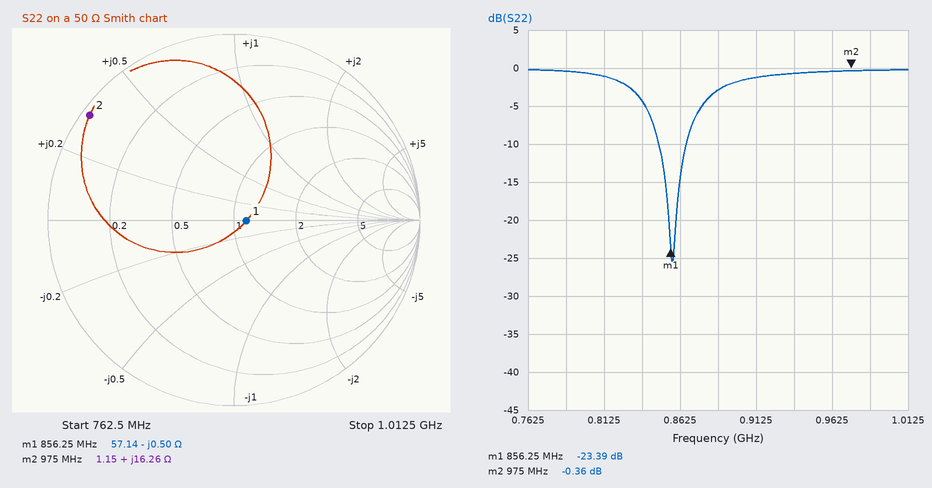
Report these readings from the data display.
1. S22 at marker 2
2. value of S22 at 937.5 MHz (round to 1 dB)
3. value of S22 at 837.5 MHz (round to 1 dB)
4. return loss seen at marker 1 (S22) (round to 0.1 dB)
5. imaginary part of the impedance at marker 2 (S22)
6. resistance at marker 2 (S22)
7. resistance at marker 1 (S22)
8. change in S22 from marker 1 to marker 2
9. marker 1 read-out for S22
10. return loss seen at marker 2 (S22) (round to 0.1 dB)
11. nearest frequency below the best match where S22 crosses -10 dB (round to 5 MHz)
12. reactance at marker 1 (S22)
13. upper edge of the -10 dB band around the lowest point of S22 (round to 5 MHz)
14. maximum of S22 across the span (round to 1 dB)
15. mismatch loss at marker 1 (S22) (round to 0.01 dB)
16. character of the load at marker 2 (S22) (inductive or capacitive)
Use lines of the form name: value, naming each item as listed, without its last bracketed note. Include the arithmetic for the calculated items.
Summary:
S22 at marker 2: -0.36 dB
value of S22 at 937.5 MHz: -1 dB
value of S22 at 837.5 MHz: -4 dB
return loss seen at marker 1 (S22): 23.5 dB
imaginary part of the impedance at marker 2: +16.26 Ω
resistance at marker 2: 1.15 Ω
resistance at marker 1: 57.14 Ω
change in S22 from marker 1 to marker 2: -0.36 − (-23.39) = 23.03 dB
marker 1 read-out for S22: -23.39 dB
return loss seen at marker 2 (S22): 0.4 dB
nearest frequency below the best match where S22 crosses -10 dB: 850 MHz
reactance at marker 1: -0.50 Ω
upper edge of the -10 dB band around the lowest point of S22: 865 MHz
maximum of S22 across the span: 0 dB
mismatch loss at marker 1 (S22): −10 log10(1 − 10^(-23.39/10)) ≈ 0.02 dB
character of the load at marker 2 (S22): inductive
